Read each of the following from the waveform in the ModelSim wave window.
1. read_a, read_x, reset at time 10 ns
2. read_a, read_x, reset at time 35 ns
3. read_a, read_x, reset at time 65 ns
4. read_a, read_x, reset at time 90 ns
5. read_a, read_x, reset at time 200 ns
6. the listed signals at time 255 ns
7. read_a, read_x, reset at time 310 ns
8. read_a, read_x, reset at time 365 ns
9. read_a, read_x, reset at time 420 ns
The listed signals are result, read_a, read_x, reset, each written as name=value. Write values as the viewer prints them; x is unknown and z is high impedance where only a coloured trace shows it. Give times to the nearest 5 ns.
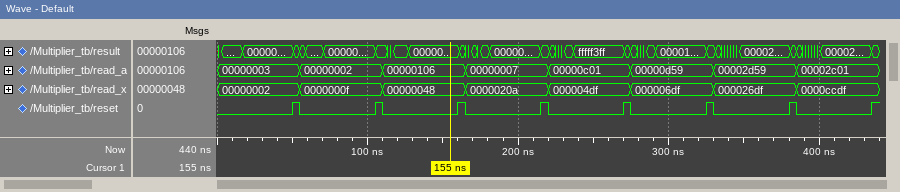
read_a=00000003, read_x=00000002, reset=0
read_a=00000003, read_x=00000002, reset=0
read_a=00000002, read_x=0000000f, reset=0
read_a=00000002, read_x=0000000f, reset=0
read_a=00000007, read_x=0000020a, reset=0
result=fffff3ff, read_a=00000c01, read_x=000004df, reset=0
read_a=00000d59, read_x=000006df, reset=0
read_a=00002d59, read_x=000026df, reset=0
read_a=00002c01, read_x=0000ccdf, reset=0
